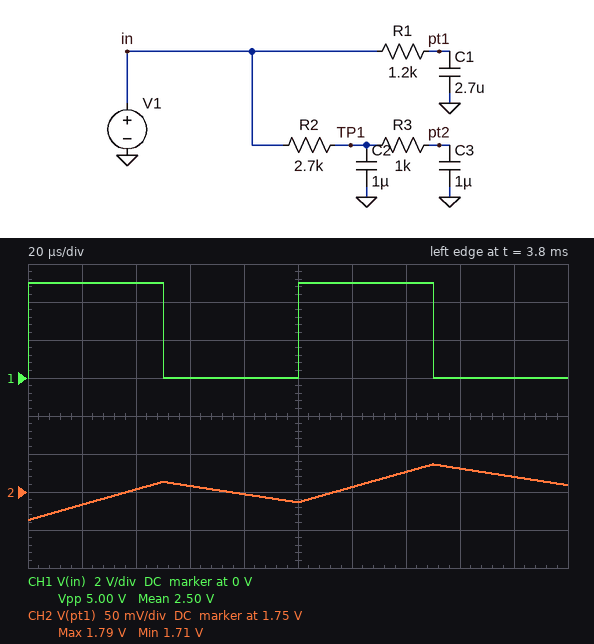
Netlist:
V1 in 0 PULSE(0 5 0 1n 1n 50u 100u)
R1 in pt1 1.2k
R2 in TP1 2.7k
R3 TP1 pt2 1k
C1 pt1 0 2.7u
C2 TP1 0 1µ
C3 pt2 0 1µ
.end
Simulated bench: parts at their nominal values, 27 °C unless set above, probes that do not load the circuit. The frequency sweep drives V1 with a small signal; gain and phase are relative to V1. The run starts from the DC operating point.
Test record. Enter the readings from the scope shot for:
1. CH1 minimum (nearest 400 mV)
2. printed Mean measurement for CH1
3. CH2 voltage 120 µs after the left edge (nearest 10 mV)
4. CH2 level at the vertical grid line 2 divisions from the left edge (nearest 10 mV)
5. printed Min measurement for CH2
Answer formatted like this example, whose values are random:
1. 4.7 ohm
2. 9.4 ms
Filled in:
1. 0 V
2. 2.50 V
3. 1.76 V
4. 1.75 V
5. 1.71 V
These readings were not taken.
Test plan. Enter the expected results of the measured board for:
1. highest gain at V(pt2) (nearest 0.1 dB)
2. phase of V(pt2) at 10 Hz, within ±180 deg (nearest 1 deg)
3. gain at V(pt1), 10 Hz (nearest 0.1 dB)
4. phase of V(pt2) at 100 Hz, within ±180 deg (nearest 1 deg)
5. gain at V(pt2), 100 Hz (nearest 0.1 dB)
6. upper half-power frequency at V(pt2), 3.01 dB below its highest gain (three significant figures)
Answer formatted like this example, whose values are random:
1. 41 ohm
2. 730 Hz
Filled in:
1. 0 dB
2. -22 deg
3. -0.2 dB
4. -91 deg
5. -12.1 dB
6. 26.6 Hz
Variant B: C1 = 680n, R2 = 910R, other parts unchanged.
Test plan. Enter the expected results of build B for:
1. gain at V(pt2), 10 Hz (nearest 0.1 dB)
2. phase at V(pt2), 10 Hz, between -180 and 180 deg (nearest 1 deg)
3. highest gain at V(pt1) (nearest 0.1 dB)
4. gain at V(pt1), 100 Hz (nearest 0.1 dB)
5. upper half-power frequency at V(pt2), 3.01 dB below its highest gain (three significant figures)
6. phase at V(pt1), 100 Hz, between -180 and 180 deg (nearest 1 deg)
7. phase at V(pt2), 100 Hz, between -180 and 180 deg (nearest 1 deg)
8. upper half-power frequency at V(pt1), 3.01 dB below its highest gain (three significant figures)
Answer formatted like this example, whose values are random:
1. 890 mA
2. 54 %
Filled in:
1. -0.1 dB
2. -10 deg
3. 0 dB
4. -1.0 dB
5. 63.6 Hz
6. -27 deg
7. -70 deg
8. 195 Hz
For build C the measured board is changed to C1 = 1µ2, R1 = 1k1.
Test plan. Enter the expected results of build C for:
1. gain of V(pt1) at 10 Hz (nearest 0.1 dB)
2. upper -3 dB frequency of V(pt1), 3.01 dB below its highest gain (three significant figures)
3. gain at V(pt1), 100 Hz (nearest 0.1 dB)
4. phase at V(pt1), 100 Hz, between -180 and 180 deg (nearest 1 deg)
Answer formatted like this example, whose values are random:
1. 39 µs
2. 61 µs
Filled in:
1. 0 dB
2. 121 Hz
3. -2.3 dB
4. -40 deg
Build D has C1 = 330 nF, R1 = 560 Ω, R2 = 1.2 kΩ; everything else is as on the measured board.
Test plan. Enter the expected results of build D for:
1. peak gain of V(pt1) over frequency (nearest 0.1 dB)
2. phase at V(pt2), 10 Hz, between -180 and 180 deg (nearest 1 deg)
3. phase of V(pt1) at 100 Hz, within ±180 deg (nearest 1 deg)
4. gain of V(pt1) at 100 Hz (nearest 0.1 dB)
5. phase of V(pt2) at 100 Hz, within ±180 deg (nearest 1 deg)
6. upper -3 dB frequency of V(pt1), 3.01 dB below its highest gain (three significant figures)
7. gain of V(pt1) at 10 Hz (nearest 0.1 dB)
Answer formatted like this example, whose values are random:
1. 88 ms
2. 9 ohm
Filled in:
1. 0 dB
2. -12 deg
3. -7 deg
4. -0.1 dB
5. -76 deg
6. 861 Hz
7. 0 dB
